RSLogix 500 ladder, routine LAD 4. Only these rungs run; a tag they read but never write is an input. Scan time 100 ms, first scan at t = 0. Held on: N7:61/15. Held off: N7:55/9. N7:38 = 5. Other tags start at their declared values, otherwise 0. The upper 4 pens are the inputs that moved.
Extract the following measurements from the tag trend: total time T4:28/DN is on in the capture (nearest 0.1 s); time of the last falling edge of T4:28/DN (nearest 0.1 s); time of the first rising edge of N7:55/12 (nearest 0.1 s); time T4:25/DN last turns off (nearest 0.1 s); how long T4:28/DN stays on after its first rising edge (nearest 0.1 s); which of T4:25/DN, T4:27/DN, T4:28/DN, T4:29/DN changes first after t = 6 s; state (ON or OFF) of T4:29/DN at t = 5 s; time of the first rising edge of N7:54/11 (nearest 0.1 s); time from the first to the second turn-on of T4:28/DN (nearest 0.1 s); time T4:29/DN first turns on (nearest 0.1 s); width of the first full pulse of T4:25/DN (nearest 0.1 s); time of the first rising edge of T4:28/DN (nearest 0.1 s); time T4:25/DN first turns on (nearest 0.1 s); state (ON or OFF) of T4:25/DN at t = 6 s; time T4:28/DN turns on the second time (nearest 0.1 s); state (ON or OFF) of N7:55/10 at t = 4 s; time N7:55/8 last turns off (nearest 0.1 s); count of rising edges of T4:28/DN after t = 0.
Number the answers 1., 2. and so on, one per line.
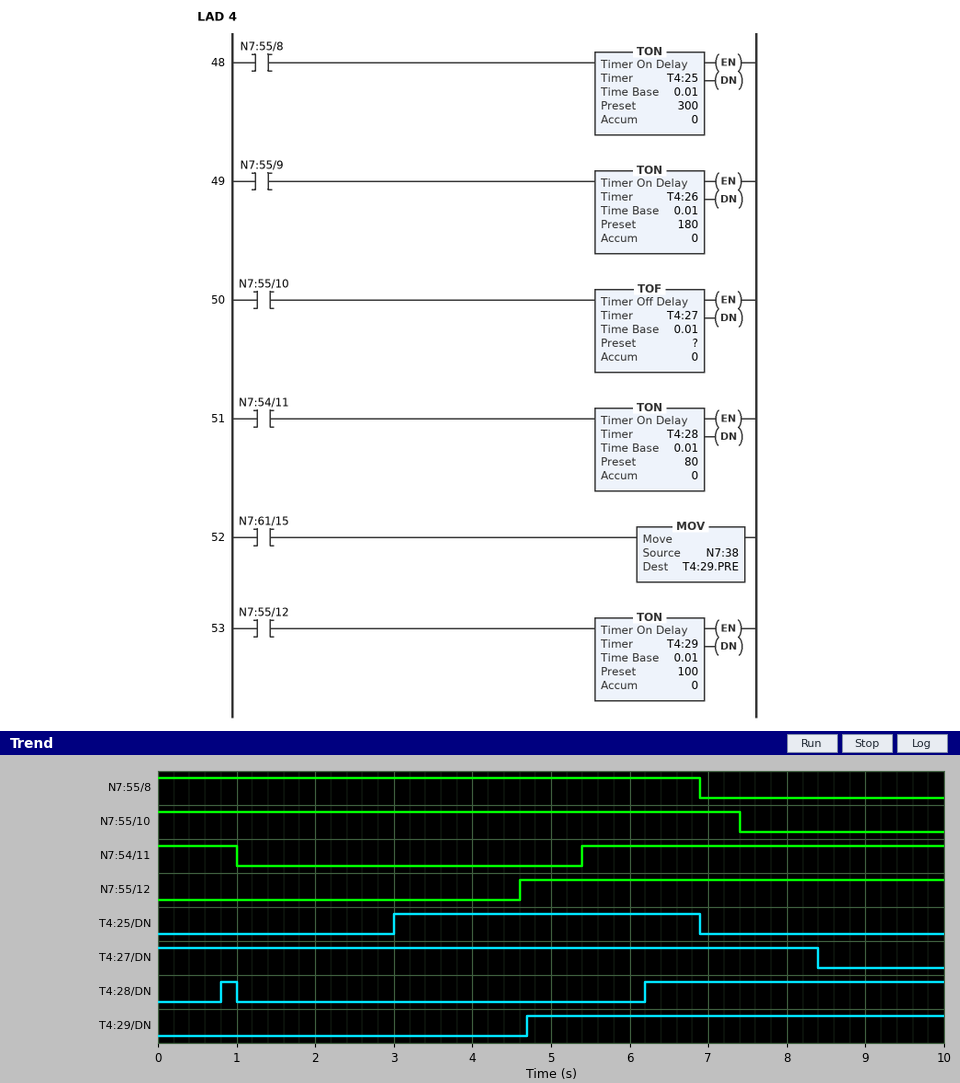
1. 4.0 s
2. 1.0 s
3. 4.6 s
4. 6.9 s
5. 0.2 s
6. T4:28/DN
7. ON
8. 5.4 s
9. 5.4 s
10. 4.7 s
11. 3.9 s
12. 0.8 s
13. 3.0 s
14. ON
15. 6.2 s
16. ON
17. 6.9 s
18. 2
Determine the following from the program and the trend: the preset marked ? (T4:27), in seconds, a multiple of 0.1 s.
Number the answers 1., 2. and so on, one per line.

1. 1.0 s
